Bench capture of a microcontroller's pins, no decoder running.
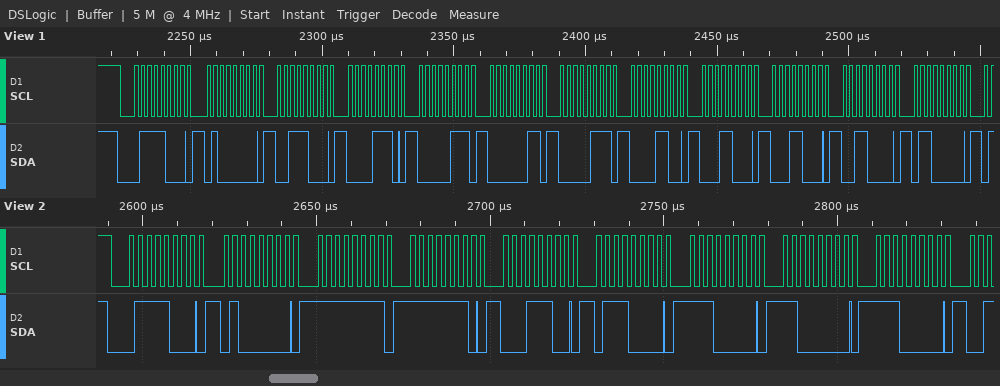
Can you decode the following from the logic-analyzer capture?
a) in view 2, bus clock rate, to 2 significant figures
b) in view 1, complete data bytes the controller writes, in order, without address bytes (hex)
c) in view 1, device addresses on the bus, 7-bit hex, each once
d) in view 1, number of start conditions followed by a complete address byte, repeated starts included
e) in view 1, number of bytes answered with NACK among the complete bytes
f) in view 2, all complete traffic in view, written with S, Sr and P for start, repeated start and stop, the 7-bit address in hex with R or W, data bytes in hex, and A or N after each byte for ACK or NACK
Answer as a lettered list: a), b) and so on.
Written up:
a) 400 kHz
b) 40 38 0E 07 03 07 0C 18 18 30 60
c) 0x3C
d) 1
e) 0
f) S 3CW A 40 A FF A FE A 1C A 70 A E0 A C0 A E0 A
